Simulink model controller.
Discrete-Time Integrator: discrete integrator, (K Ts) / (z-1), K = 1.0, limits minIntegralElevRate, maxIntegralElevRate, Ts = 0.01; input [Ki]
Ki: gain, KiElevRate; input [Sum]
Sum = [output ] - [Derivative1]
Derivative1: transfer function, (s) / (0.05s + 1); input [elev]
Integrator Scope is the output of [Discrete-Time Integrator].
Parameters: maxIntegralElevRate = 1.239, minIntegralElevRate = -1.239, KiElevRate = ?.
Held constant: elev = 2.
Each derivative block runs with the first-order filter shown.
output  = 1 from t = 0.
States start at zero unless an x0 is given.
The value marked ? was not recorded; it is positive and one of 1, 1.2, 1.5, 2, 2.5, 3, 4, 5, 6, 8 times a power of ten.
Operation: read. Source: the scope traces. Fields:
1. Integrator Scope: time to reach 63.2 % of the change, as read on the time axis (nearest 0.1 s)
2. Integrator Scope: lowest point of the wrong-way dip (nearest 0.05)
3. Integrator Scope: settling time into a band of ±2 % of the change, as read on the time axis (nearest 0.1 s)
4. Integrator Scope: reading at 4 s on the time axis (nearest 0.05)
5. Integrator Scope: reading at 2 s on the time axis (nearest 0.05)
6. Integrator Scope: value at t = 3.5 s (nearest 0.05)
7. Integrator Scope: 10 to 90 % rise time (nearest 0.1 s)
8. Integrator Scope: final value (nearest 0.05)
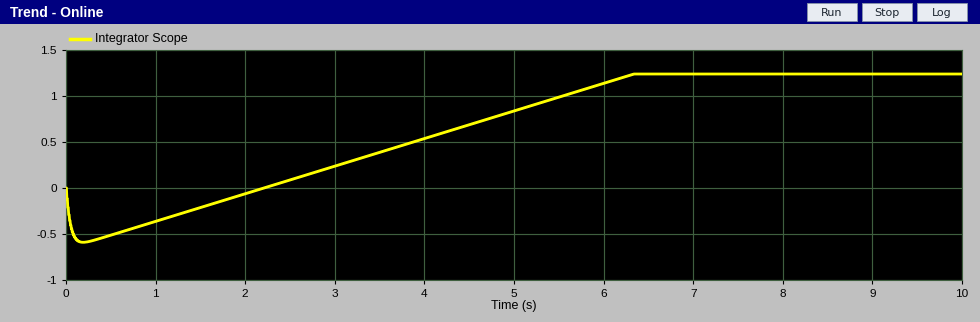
4.8 s
-0.60
6.3 s
0.55
-0.05
0.40
3.3 s
1.25
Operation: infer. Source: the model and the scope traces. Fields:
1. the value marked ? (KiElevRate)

0.3
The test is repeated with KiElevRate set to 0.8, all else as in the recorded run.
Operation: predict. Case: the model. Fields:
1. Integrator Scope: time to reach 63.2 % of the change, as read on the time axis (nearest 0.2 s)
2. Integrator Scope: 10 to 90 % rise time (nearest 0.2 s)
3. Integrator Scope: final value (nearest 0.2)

2.8 s
1.2 s
1.2
